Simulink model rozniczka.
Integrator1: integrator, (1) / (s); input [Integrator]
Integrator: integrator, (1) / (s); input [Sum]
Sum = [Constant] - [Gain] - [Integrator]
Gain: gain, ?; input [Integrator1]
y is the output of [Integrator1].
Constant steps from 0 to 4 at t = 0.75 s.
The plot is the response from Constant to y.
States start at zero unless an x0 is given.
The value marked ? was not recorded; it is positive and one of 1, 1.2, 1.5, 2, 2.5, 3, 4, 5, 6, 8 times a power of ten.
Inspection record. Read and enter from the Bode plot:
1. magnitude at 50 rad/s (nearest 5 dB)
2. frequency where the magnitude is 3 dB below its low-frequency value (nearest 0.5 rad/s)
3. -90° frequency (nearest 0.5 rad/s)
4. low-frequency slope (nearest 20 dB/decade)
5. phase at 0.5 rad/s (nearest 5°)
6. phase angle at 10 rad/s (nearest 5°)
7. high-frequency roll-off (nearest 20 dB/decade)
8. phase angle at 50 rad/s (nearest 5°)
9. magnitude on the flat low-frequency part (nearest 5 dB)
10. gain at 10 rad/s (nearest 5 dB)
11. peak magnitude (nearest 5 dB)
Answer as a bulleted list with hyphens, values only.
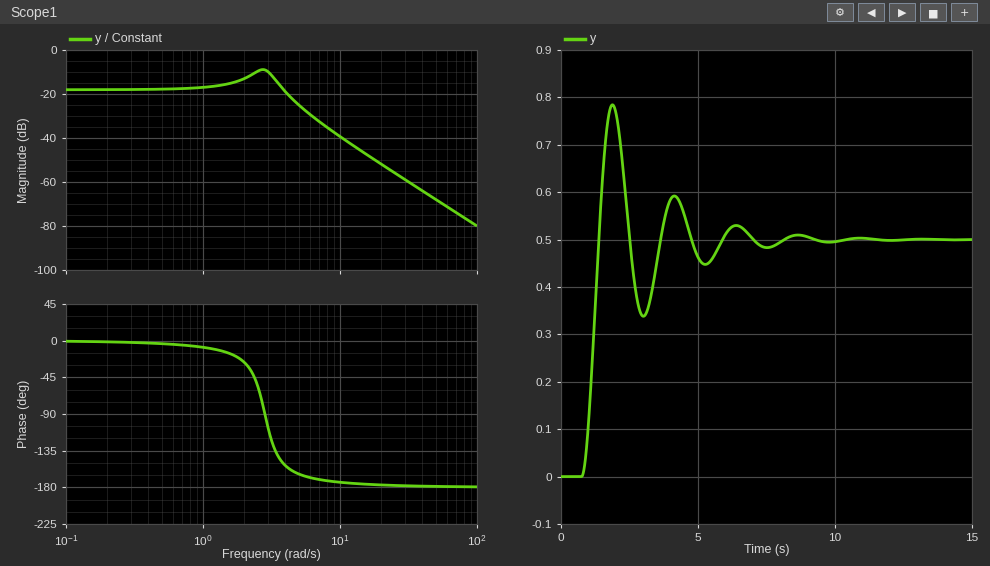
- -70 dB
- 4.5 rad/s
- 3.0 rad/s
- 0 dB/decade
- -5°
- -175°
- -40 dB/decade
- -180°
- -20 dB
- -40 dB
- -10 dB
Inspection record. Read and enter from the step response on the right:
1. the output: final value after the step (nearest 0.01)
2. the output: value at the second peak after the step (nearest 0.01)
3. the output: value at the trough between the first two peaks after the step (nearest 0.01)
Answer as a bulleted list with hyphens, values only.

- 0.50
- 0.59
- 0.34
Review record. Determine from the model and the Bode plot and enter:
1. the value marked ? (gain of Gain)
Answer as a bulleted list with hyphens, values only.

- 8
